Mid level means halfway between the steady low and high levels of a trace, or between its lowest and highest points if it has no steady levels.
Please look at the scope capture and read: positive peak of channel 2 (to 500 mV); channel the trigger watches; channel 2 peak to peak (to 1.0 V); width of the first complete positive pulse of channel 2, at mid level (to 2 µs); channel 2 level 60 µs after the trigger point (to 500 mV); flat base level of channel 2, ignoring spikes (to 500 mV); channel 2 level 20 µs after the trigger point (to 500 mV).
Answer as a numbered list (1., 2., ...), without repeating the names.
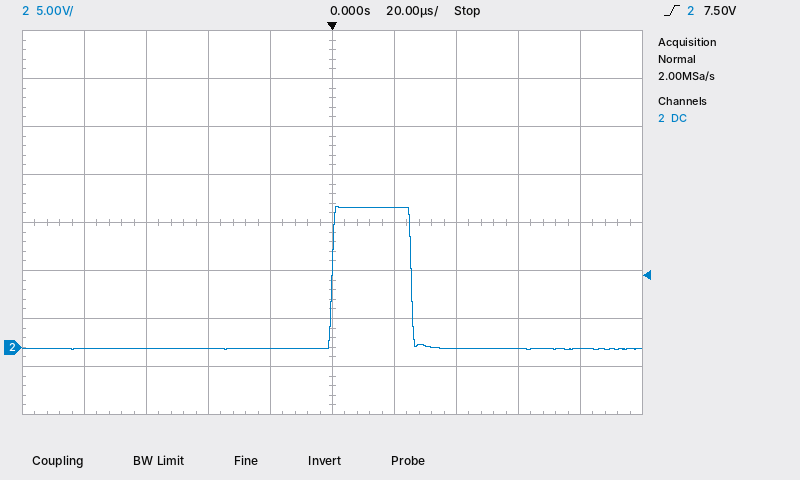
1. 14.5 V
2. channel 2
3. 15.0 V
4. 26 µs
5. 0.0 V
6. 0.0 V
7. 14.5 V
